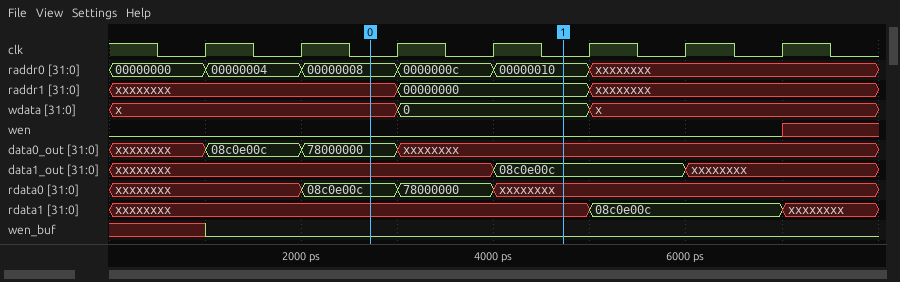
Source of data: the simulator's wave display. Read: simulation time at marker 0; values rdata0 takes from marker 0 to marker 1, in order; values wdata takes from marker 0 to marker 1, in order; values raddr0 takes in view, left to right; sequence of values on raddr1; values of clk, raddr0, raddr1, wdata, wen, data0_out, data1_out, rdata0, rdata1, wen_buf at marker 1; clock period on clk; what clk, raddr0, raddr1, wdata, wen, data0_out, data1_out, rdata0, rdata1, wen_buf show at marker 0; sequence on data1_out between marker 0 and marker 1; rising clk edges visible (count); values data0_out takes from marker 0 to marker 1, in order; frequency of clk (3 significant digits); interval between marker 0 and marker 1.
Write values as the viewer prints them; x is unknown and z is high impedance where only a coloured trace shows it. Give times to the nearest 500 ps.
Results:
2500 ps
08c0e00c, 78000000, xxxxxxxx
x, 0
00000000, 00000004, 00000008, 0000000c, 00000010, xxxxxxxx
xxxxxxxx, 00000000, xxxxxxxx
clk=0, raddr0=00000010, raddr1=00000000, wdata=0, wen=0, data0_out=xxxxxxxx, data1_out=08c0e00c, rdata0=xxxxxxxx, rdata1=xxxxxxxx, wen_buf=0
1000 ps
clk=0, raddr0=00000008, raddr1=xxxxxxxx, wdata=x, wen=0, data0_out=78000000, data1_out=xxxxxxxx, rdata0=08c0e00c, rdata1=xxxxxxxx, wen_buf=0
xxxxxxxx, 08c0e00c
7
78000000, xxxxxxxx
1.00 GHz
2000 ps
